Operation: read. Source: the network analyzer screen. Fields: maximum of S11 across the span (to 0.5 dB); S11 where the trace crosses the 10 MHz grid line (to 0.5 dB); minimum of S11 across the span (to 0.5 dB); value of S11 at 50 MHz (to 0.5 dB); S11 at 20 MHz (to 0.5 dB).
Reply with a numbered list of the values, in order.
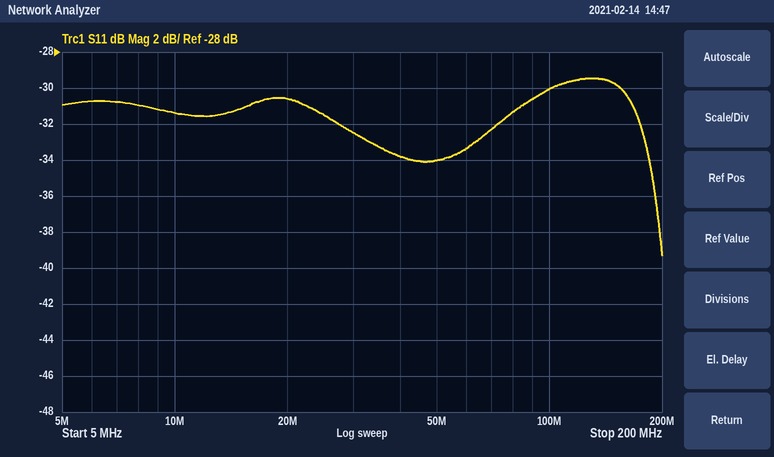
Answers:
1. -29.5 dB
2. -31.5 dB
3. -39.5 dB
4. -34.0 dB
5. -30.5 dB
